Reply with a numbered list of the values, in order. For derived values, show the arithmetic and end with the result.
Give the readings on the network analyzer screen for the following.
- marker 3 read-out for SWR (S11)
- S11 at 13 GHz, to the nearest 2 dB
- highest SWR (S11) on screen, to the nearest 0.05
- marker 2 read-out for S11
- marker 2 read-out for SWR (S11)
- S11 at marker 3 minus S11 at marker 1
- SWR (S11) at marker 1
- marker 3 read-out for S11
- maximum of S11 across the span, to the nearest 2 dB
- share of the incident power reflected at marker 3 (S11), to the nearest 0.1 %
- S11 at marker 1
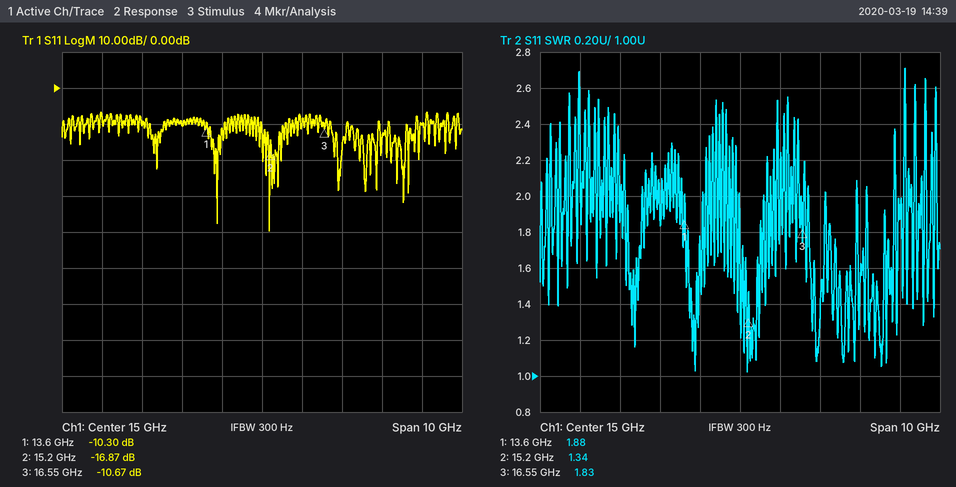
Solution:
1. 1.83
2. -10 dB
3. 2.70
4. -16.87 dB
5. 1.34
6. -10.67 − (-10.3) = -0.37 dB
7. 1.88
8. -10.67 dB
9. -6 dB
10. 10^(-10.67/10) ≈ 8.6 %
11. -10.30 dB
